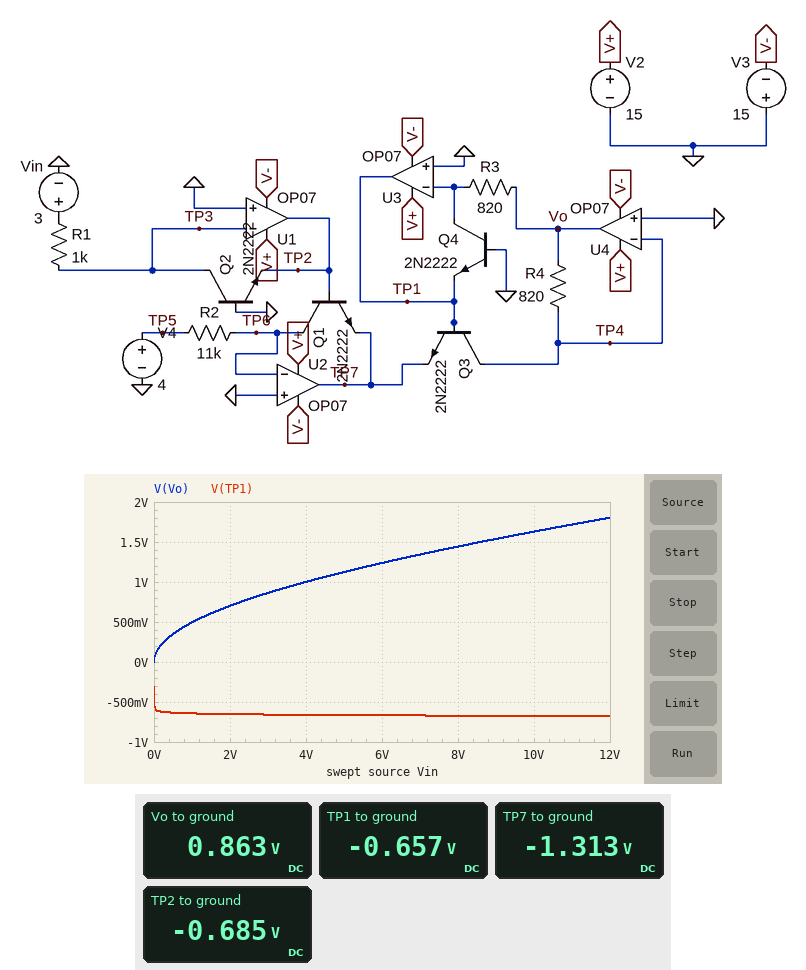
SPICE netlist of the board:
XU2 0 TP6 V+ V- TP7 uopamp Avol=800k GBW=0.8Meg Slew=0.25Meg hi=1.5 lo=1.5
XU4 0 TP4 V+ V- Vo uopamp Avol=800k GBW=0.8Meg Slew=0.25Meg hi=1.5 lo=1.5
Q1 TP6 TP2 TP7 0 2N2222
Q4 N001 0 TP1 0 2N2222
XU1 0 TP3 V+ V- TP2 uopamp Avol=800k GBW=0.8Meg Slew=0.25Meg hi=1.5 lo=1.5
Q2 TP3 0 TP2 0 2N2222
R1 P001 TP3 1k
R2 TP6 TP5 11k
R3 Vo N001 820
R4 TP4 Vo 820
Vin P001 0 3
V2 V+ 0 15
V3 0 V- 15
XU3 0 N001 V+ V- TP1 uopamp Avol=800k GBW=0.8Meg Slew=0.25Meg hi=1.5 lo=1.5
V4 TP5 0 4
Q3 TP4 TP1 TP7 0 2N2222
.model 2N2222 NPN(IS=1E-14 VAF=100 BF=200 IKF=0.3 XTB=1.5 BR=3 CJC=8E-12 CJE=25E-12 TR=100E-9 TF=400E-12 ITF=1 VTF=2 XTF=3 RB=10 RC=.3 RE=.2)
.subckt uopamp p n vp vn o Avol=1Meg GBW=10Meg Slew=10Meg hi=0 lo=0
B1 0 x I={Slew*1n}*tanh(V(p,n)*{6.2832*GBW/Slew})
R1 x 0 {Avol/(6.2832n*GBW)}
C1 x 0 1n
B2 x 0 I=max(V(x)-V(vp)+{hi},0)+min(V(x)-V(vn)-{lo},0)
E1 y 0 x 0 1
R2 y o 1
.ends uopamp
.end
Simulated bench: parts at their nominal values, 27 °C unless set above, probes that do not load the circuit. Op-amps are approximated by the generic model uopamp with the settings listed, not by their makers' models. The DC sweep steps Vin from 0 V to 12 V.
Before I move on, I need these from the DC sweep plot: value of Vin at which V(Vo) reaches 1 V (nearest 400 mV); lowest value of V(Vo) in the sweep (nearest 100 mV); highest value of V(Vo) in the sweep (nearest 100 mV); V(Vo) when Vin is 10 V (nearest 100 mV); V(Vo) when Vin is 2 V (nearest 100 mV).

4.0 V
0 V
1.8 V
1.6 V
700 mV
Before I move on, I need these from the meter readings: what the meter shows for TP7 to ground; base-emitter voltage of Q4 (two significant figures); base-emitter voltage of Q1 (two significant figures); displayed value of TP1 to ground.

-1.313 V
660 mV
630 mV
-0.657 V
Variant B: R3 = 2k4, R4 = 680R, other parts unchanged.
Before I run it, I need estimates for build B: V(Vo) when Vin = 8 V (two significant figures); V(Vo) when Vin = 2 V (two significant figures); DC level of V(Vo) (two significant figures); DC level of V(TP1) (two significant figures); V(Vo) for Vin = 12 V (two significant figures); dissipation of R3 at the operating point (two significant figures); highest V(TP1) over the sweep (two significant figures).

2.2 V
1.1 V
1.3 V
-640 mV
2.8 V
750 µW
-300 mV
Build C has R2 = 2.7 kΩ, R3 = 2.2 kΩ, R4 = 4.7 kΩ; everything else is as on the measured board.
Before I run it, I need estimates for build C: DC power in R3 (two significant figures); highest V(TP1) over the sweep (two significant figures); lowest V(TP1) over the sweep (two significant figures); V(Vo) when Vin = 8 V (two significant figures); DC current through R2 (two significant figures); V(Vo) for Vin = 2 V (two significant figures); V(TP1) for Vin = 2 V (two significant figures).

21 mW
-340 mV
-700 mV
11 V
1.5 mA
5.5 V
-680 mV
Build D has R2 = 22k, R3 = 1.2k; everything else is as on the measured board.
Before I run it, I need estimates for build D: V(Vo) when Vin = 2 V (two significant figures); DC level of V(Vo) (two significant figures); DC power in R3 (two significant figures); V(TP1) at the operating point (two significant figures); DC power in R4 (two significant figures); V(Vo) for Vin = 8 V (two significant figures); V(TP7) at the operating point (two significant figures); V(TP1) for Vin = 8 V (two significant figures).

600 mV
740 mV
460 µW
-640 mV
670 µW
1.2 V
-1.3 V
-660 mV
